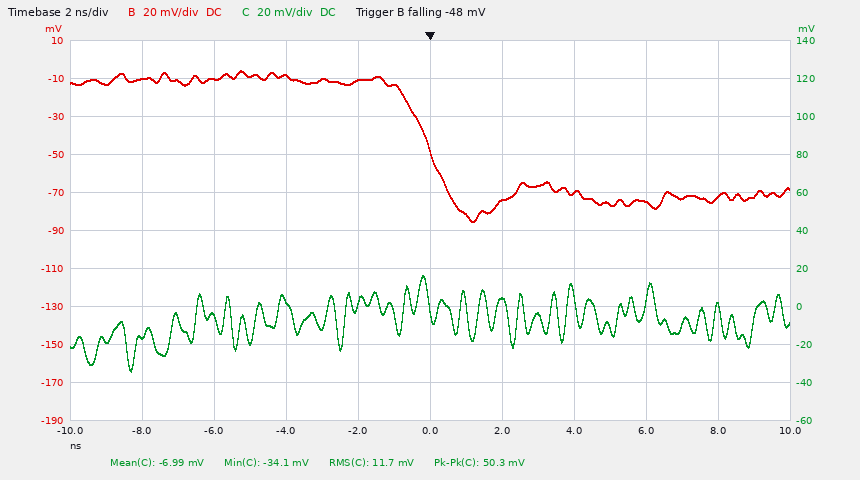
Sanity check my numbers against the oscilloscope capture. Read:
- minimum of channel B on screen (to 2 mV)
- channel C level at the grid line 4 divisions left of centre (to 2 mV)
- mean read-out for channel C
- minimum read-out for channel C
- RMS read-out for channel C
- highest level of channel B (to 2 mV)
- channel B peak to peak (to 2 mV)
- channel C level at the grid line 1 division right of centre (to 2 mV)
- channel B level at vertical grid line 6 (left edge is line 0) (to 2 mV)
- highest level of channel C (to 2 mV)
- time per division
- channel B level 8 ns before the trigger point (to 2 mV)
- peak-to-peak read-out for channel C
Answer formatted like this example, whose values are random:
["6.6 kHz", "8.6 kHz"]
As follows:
["-86 mV", "-16 mV", "-6.99 mV", "-34.1 mV", "11.7 mV", "-6 mV", "80 mV", "4 mV", "-74 mV", "16 mV", "2 ns", "-10 mV", "50.3 mV"]
